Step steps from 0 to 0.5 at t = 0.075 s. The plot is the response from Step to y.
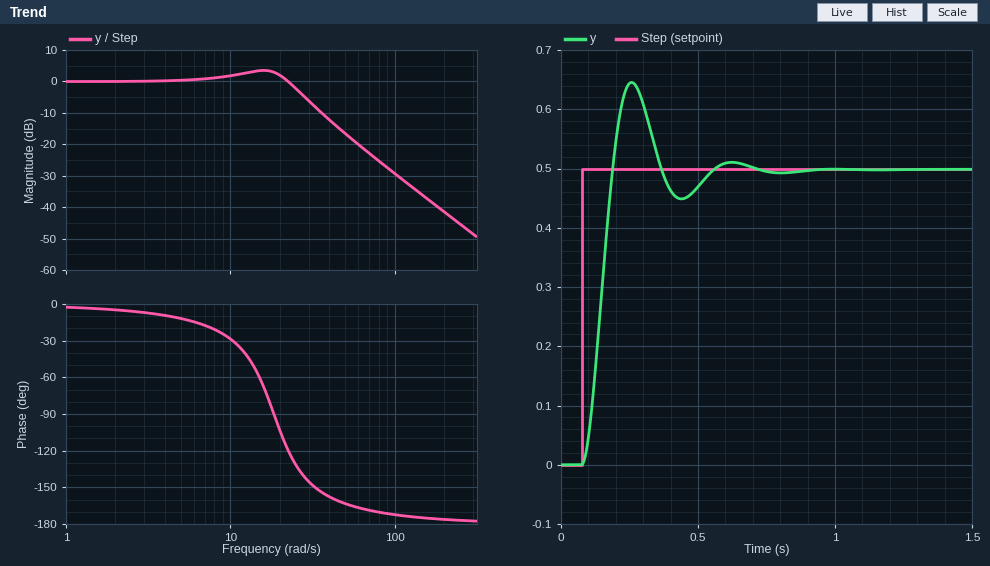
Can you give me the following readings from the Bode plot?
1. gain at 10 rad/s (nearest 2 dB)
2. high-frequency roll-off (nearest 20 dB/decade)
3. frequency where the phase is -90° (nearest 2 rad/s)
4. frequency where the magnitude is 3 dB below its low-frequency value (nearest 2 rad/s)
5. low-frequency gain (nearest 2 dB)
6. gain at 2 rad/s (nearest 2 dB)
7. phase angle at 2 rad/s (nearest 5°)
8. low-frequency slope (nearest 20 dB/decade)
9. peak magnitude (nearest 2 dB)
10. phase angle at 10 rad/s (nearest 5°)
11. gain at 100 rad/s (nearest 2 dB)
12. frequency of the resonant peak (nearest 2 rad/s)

2 dB
-40 dB/decade
18 rad/s
26 rad/s
0 dB
0 dB
-5°
0 dB/decade
4 dB
-30°
-30 dB
16 rad/s
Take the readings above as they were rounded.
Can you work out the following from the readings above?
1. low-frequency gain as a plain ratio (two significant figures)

1.0
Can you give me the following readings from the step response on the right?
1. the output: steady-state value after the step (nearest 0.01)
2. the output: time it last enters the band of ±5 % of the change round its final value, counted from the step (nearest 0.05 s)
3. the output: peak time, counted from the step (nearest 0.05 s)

0.50
0.45 s
0.20 s
